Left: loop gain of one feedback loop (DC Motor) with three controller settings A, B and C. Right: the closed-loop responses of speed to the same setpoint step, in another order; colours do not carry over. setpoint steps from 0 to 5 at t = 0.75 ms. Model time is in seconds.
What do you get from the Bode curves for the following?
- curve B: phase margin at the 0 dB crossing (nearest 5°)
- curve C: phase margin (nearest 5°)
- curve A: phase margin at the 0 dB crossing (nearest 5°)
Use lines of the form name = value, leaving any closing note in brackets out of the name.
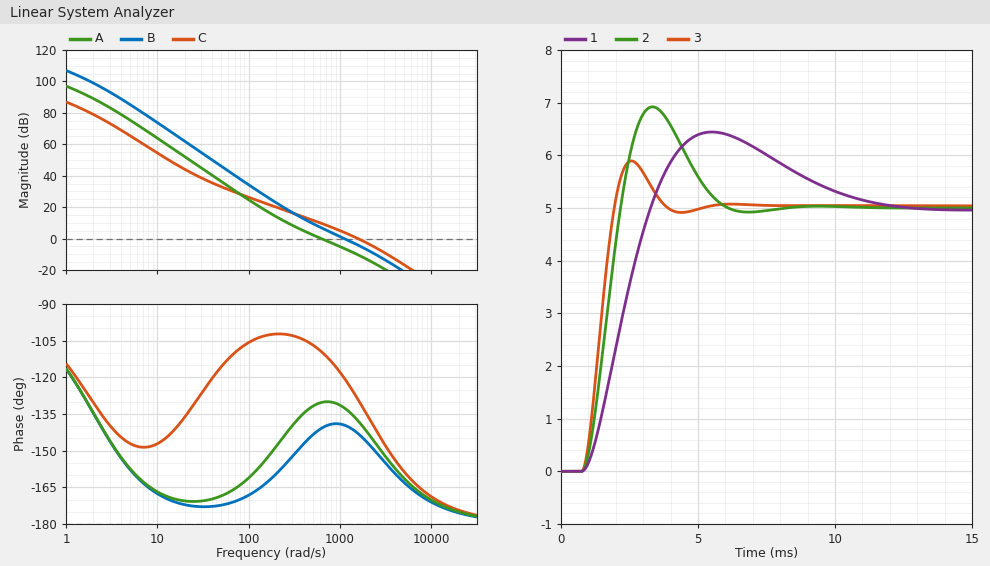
curve B: phase margin at the 0 dB crossing = 40°
curve C: phase margin = 50°
curve A: phase margin at the 0 dB crossing = 50°
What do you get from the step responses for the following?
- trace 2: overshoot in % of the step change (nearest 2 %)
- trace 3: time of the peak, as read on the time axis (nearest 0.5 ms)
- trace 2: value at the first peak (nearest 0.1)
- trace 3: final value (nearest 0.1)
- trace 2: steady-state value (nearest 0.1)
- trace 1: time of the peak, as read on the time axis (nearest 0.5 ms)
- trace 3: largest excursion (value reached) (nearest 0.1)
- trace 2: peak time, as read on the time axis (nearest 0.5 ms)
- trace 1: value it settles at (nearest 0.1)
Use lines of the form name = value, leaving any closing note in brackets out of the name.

trace 2: overshoot in % of the step change = 38 %
trace 3: time of the peak, as read on the time axis = 2.5 ms
trace 2: value at the first peak = 6.9
trace 3: final value = 5.0
trace 2: steady-state value = 5.0
trace 1: time of the peak, as read on the time axis = 5.5 ms
trace 3: largest excursion (value reached) = 5.9
trace 2: peak time, as read on the time axis = 3.5 ms
trace 1: value it settles at = 5.0
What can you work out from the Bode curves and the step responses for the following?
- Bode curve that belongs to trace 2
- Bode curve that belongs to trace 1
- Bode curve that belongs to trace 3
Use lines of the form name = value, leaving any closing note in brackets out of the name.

Bode curve that belongs to trace 2 = B
Bode curve that belongs to trace 1 = A
Bode curve that belongs to trace 3 = C
